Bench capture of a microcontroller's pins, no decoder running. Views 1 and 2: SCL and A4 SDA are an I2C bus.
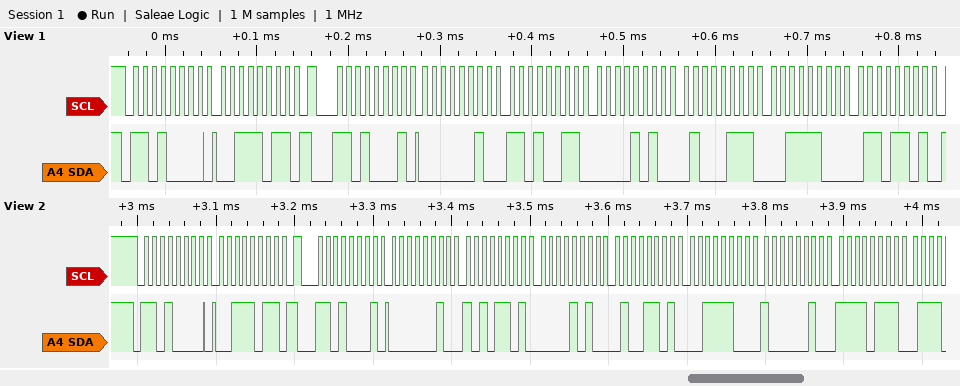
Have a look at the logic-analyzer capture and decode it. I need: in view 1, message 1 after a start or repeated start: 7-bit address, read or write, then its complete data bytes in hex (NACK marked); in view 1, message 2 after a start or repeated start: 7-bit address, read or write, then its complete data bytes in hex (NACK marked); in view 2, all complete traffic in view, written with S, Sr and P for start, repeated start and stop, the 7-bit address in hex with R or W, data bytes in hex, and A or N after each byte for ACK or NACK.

0x68 write: 3B
0x68 read: 02 D3 0A 47 3C 6D
S 68W A 3B A Sr 68R A 02 A AD A 0A A 4D A 3C A 82 A F7 A
